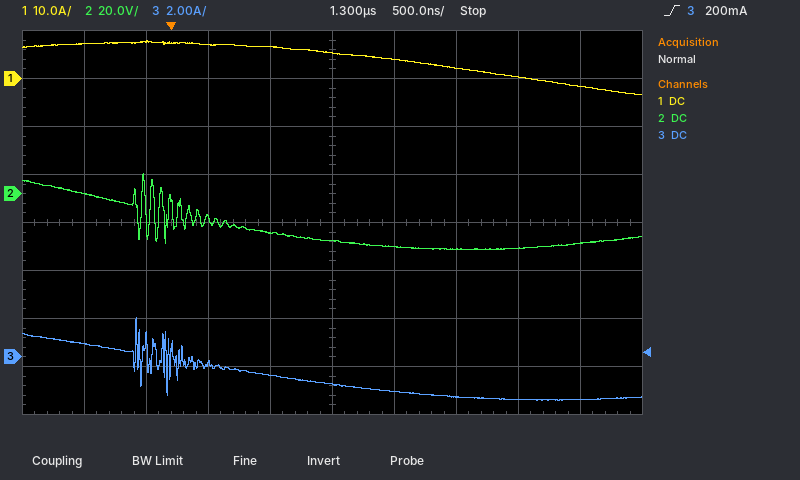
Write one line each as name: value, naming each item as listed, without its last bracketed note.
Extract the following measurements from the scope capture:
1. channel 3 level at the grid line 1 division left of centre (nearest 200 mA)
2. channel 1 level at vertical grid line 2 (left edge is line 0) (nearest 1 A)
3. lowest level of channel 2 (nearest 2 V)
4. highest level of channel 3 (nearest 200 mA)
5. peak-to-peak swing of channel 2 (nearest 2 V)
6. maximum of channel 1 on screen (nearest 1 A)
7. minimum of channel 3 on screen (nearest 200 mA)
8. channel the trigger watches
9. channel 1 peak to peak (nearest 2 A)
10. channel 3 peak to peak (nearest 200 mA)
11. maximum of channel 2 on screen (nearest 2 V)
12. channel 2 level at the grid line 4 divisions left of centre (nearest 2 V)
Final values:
channel 3 level at the grid line 1 division left of centre: -800 mA
channel 1 level at vertical grid line 2 (left edge is line 0): 8 A
lowest level of channel 2: -24 V
highest level of channel 3: 1.6 A
peak-to-peak swing of channel 2: 32 V
maximum of channel 1 on screen: 8 A
minimum of channel 3 on screen: -1.8 A
channel the trigger watches: channel 3
channel 1 peak to peak: 12 A
channel 3 peak to peak: 3.4 A
maximum of channel 2 on screen: 8 V
channel 2 level at the grid line 4 divisions left of centre: 0 V
